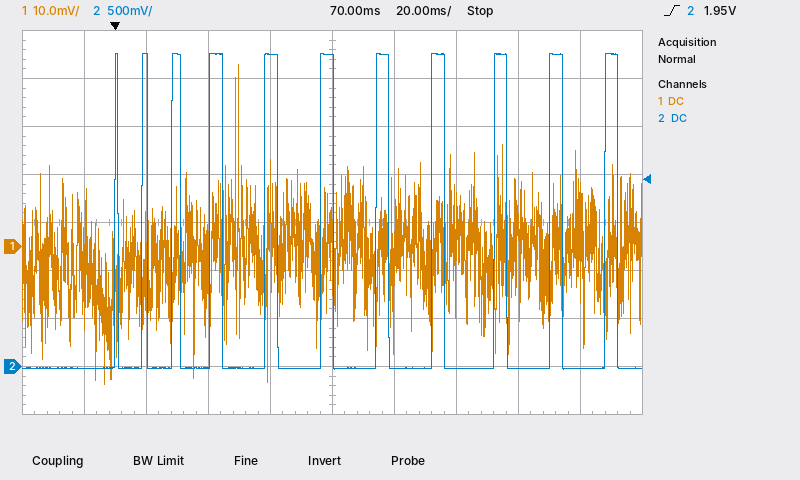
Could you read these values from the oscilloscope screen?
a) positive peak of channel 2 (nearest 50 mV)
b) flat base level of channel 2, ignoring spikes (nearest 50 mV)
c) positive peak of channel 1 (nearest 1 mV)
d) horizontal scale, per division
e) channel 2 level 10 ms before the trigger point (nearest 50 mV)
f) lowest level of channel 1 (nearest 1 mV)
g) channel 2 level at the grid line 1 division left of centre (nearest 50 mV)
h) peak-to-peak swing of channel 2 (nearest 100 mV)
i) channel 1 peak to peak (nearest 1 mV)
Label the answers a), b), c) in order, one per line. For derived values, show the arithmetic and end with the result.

a) 3.25 V
b) 0 mV
c) 38 mV
d) 20 ms
e) 0 mV
f) -29 mV
g) 3.25 V
h) 3.30 V
i) 38 mV − (-29 mV) = 67 mV
